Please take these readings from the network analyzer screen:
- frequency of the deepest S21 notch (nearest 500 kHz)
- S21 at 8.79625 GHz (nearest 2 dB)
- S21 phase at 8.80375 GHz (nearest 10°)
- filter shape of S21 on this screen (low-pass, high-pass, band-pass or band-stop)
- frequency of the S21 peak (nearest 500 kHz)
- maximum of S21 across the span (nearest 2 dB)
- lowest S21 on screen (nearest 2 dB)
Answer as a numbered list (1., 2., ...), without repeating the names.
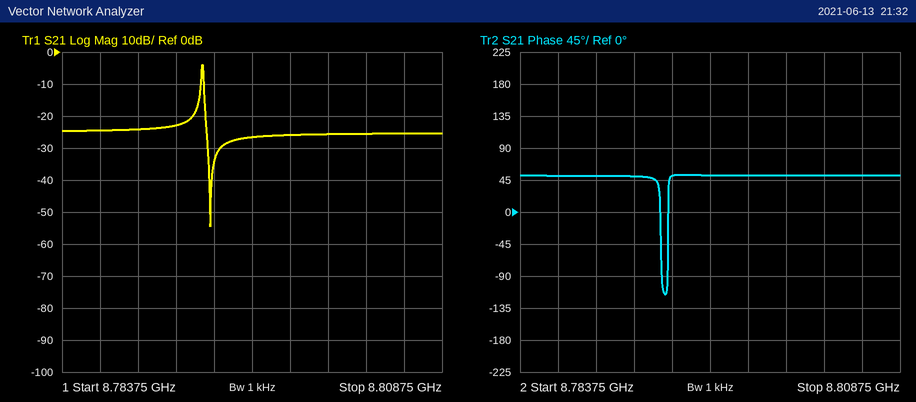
1. 8.7935 GHz
2. -26 dB
3. 50°
4. band-pass
5. 8.7930 GHz
6. -4 dB
7. -54 dB
